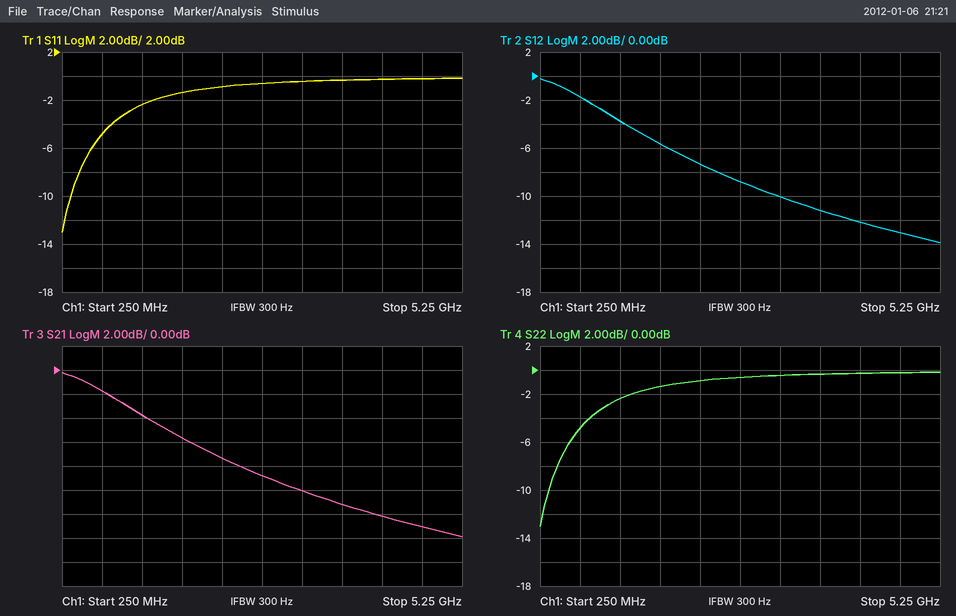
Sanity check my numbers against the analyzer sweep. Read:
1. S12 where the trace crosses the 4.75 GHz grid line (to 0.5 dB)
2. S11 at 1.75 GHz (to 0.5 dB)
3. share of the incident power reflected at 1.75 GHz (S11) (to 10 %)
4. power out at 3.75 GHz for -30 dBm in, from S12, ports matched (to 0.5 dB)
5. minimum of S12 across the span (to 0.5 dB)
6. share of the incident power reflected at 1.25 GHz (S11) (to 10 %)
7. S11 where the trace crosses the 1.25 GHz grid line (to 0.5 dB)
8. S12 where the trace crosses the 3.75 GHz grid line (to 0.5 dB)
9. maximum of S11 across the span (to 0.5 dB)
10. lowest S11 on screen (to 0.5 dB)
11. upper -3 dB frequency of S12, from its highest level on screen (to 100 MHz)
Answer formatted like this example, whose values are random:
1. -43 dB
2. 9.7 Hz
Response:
1. -13.0 dB
2. -1.5 dB
3. 70 %
4. -41.0 dBm
5. -14.0 dB
6. 60 %
7. -2.5 dB
8. -11.0 dB
9. 0.0 dB
10. -13.0 dB
11. 1.1 GHz
